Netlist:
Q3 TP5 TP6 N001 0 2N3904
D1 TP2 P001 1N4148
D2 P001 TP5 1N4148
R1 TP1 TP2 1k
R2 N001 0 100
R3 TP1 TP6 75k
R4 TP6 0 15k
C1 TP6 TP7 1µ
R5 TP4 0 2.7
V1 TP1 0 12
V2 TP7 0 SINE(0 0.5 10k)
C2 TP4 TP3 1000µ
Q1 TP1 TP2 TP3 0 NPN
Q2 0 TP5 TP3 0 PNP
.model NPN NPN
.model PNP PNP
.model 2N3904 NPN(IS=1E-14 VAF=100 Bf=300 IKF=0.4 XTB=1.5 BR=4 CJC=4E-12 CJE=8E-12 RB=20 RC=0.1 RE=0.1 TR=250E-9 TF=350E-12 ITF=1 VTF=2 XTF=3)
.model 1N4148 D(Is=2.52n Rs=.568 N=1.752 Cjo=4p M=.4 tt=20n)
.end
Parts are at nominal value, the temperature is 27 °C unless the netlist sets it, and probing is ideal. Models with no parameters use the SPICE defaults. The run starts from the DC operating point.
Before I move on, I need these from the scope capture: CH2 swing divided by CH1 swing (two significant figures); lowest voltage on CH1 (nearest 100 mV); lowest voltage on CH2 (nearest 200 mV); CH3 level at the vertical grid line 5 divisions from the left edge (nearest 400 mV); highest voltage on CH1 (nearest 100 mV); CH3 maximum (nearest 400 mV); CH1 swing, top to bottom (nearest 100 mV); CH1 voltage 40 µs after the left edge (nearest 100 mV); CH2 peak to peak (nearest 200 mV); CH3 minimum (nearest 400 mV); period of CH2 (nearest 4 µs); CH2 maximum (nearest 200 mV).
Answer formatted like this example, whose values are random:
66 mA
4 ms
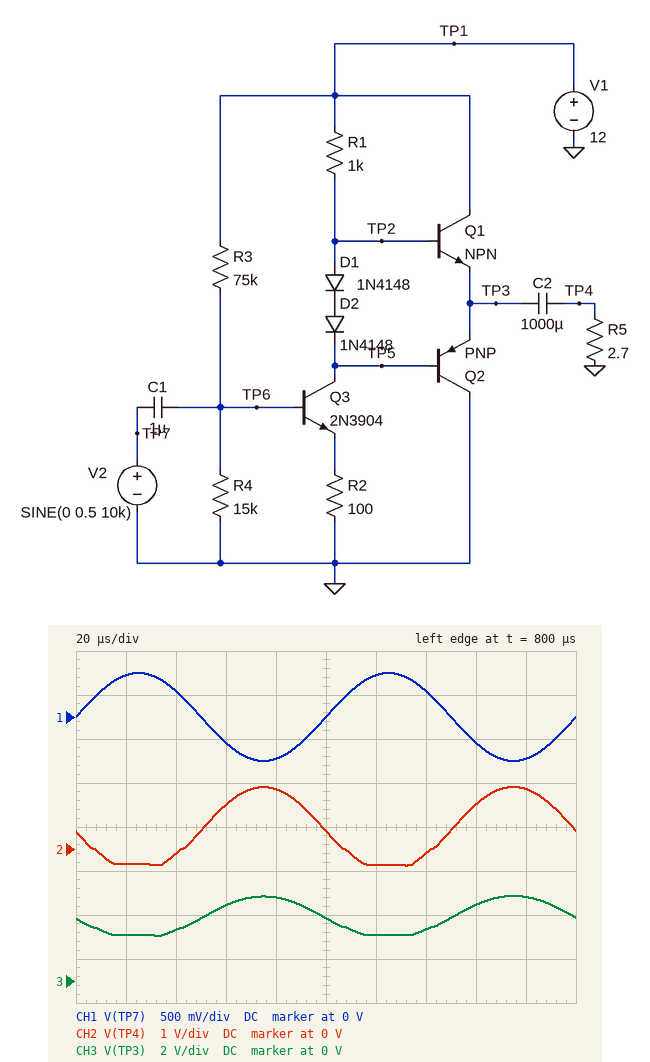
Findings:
1.8
-500 mV
-400 mV
2.8 V
500 mV
4.0 V
1.0 V
300 mV
1.8 V
2.0 V
100 µs
1.4 V
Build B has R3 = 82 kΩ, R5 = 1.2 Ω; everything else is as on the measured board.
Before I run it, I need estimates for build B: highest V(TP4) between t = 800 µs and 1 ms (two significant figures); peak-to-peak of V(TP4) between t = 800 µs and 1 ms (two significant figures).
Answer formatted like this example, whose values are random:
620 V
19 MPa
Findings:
490 mV
980 mV
